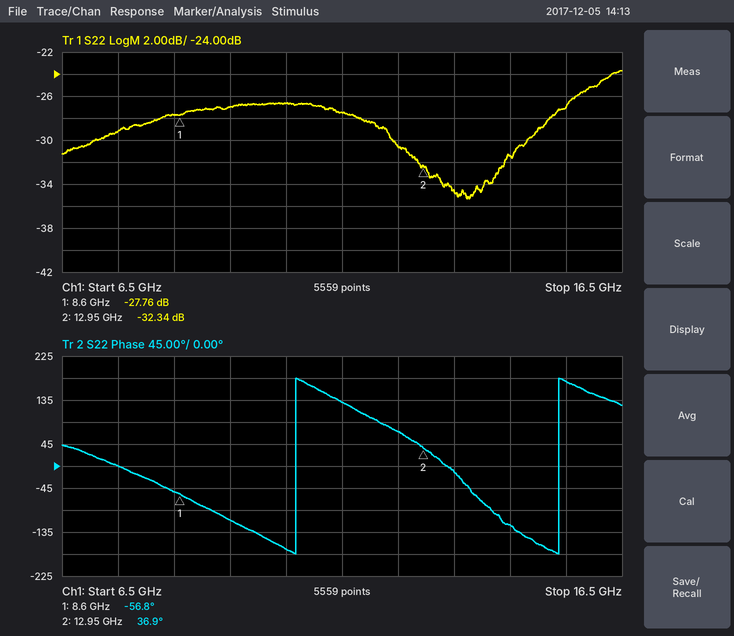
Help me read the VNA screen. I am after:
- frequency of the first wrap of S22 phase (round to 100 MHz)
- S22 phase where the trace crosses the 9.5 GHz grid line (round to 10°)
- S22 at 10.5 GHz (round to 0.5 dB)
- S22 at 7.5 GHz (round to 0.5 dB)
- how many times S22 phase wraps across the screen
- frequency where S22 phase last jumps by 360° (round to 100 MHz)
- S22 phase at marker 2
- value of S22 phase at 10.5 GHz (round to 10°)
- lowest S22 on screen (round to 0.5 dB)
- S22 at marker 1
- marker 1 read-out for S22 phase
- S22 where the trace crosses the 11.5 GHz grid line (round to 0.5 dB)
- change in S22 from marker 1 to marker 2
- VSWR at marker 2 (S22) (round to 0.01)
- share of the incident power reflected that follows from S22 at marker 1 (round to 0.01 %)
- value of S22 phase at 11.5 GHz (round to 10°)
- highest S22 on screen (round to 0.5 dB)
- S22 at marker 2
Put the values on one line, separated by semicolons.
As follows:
10.7 GHz; -110°; -26.5 dB; -29.0 dB; 2; 15.4 GHz; 36.9°; -170°; -35.5 dB; -27.76 dB; -56.8°; -27.5 dB; -4.58 dB; 1.05; 0.17 %; 130°; -23.5 dB; -32.34 dB
